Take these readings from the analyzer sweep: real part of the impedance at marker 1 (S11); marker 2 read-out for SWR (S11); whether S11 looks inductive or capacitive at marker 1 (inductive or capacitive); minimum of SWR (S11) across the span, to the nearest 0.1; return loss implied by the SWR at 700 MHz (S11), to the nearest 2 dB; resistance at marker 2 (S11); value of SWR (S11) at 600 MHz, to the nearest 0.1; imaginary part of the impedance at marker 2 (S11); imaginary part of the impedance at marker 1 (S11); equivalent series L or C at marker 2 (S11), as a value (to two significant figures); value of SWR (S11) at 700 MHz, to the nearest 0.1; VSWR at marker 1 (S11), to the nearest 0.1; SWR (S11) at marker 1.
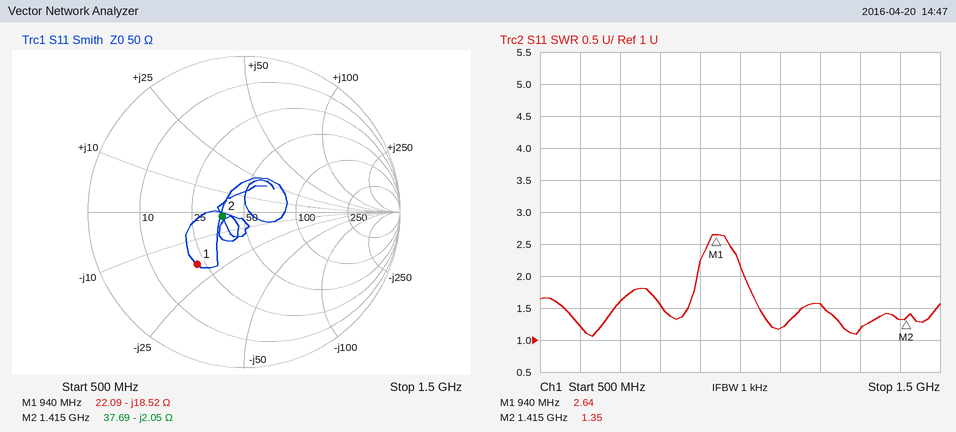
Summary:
22.09 Ω
1.35
capacitive
1.1
12 dB
37.69 Ω
1.2
-2.05 Ω
-18.52 Ω
55 pF
1.6
2.6
2.64
